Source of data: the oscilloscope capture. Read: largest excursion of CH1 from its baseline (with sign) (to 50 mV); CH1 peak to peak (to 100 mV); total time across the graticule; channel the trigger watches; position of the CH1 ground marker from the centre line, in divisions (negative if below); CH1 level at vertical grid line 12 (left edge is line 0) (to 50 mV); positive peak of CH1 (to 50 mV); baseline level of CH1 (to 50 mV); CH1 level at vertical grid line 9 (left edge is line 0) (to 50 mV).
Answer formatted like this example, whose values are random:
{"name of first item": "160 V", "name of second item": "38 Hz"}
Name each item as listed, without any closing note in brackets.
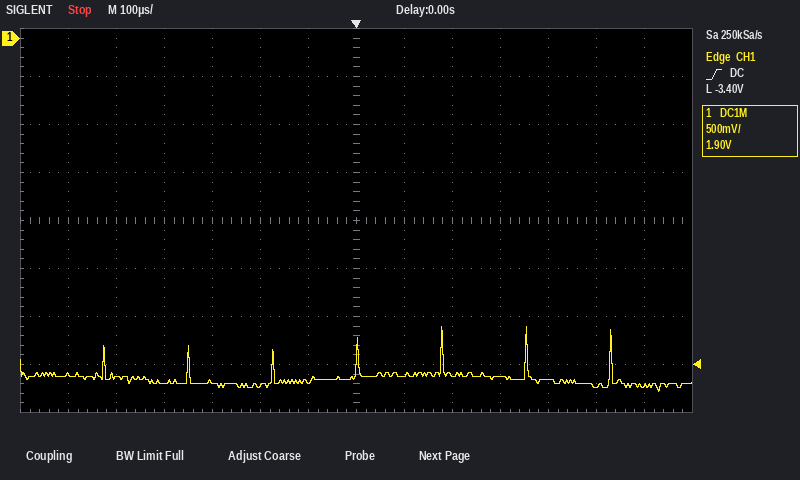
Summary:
{"largest excursion of CH1 from its baseline (with sign)": "+550 mV", "CH1 peak to peak": "700 mV", "total time across the graticule": "1.4 ms", "channel the trigger watches": "CH1", "position of the CH1 ground marker from the centre line, in divisions": "+3.8 div", "CH1 level at vertical grid line 12 (left edge is line 0)": "-3.65 V", "positive peak of CH1": "-3.00 V", "baseline level of CH1": "-3.55 V", "CH1 level at vertical grid line 9 (left edge is line 0)": "-3.50 V"}
